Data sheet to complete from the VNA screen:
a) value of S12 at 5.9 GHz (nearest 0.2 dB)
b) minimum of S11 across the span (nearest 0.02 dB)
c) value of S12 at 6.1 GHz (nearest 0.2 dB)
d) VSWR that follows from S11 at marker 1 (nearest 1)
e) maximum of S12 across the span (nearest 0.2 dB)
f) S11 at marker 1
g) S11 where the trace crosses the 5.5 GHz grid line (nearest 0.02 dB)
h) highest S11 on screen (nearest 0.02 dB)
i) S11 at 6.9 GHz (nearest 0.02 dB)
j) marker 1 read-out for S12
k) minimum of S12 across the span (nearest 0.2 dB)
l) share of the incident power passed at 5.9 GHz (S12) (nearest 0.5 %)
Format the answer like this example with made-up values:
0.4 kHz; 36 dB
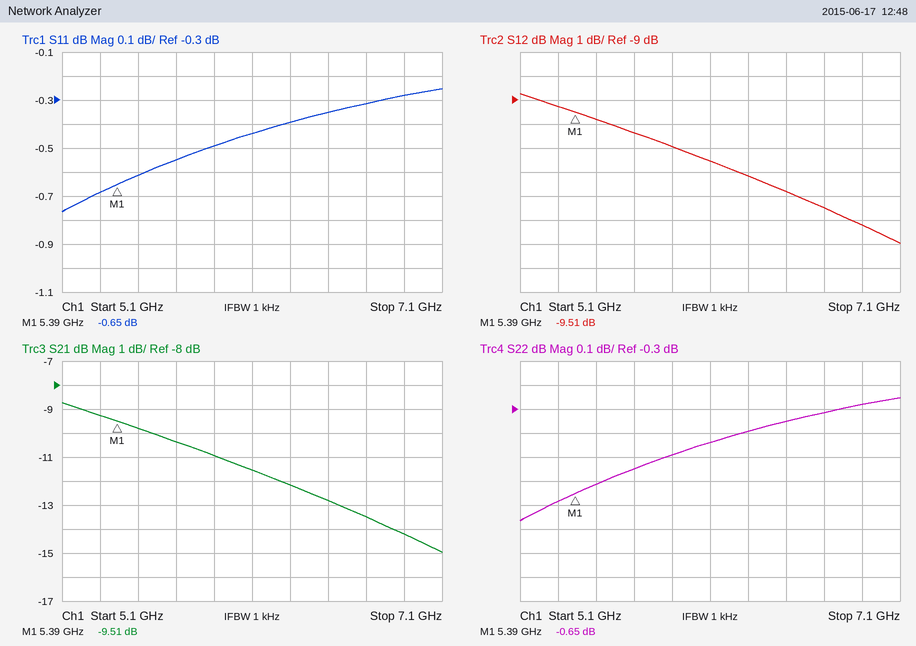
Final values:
-11.0 dB; -0.76 dB; -11.6 dB; 27; -8.8 dB; -0.65 dB; -0.62 dB; -0.26 dB; -0.28 dB; -9.51 dB; -15.0 dB; 8.0 %
